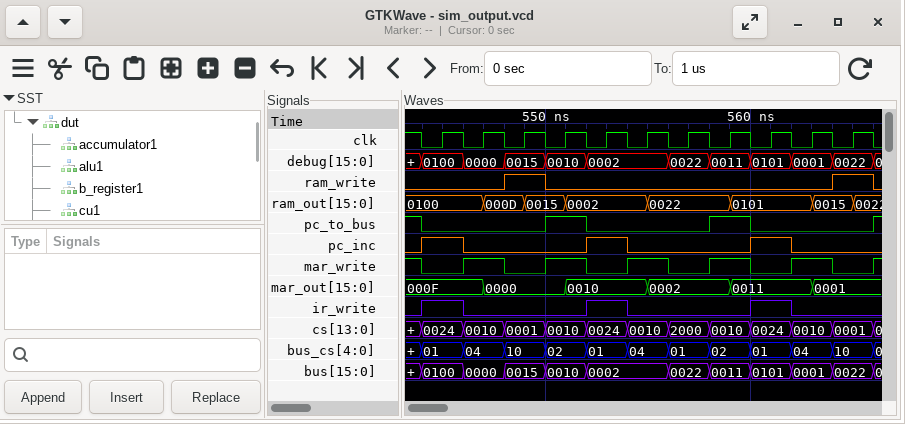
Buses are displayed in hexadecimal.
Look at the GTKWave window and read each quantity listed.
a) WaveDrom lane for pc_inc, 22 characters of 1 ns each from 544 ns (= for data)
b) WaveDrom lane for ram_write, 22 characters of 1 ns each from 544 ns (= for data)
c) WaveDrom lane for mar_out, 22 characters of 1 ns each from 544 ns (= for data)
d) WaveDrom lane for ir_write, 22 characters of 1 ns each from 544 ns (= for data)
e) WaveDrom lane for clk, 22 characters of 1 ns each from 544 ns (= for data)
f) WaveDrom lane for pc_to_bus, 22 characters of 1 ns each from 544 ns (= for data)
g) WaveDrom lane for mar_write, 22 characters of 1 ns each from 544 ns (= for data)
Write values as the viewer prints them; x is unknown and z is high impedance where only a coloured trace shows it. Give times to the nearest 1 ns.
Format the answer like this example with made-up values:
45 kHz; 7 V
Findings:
{name: 'pc_inc', wave: '1.0.....1.0.....1.0...'}; {name: 'ram_write', wave: '0...1.0.............1.'}; {name: 'mar_out', wave: '=..=...=...=...=...=..', data: '000F 0000 0010 0002 0011 0001'}; {name: 'ir_write', wave: '1.0.....1.0.....1.0...'}; {name: 'clk', wave: '0101010101010101010101'}; {name: 'pc_to_bus', wave: '0.....1.0.....1.0.....'}; {name: 'mar_write', wave: '0.1.0.1.0.1.0.1.0.1.0.'}
